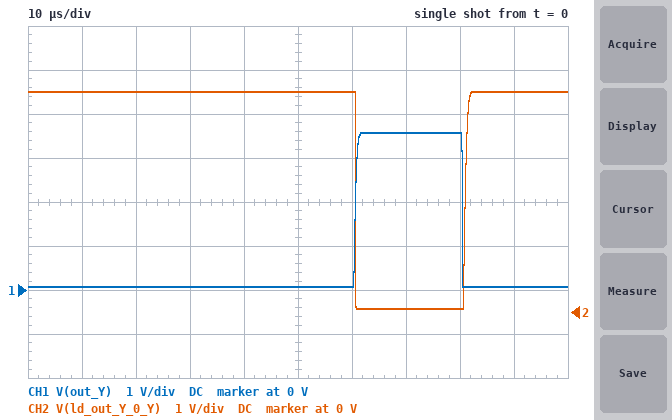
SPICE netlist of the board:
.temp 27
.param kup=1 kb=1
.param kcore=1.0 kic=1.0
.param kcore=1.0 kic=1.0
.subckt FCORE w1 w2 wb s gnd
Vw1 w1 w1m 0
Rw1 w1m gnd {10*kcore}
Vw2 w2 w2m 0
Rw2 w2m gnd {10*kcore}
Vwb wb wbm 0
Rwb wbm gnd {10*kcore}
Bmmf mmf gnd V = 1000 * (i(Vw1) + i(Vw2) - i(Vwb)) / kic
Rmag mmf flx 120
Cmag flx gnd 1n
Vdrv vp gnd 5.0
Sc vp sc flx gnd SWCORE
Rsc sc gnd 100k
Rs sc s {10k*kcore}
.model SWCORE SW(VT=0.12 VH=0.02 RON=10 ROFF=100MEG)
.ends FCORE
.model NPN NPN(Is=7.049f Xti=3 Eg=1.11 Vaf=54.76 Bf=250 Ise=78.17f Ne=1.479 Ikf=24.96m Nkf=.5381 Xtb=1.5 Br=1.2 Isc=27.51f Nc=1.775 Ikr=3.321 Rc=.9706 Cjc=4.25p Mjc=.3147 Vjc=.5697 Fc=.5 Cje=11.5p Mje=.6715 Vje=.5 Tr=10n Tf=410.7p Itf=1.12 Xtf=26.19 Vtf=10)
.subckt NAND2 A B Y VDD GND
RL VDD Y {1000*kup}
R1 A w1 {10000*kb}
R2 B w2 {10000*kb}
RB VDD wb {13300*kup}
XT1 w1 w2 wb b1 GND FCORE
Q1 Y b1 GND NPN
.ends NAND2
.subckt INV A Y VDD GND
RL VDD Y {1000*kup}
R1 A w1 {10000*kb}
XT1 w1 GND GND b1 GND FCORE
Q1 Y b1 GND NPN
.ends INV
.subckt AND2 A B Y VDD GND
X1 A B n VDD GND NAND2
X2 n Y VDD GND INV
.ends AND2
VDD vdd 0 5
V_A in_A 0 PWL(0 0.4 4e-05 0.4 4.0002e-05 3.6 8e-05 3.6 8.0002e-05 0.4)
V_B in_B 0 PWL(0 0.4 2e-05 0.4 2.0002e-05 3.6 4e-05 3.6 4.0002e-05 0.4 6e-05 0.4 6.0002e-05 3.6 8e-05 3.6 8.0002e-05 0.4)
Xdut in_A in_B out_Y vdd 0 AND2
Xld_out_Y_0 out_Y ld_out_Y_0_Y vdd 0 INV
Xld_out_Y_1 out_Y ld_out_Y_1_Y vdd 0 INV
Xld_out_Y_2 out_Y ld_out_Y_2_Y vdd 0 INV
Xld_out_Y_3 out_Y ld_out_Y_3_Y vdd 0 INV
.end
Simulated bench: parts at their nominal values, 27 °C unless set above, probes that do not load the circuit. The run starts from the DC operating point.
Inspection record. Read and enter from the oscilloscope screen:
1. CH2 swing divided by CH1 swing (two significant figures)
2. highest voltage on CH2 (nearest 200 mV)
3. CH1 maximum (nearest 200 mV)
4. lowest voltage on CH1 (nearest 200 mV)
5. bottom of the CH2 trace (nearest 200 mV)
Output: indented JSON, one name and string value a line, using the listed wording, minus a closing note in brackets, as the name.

{
  "CH2 swing divided by CH1 swing": "1.4",
  "highest voltage on CH2": "5.0 V",
  "CH1 maximum": "3.6 V",
  "lowest voltage on CH1": "0 V",
  "bottom of the CH2 trace": "0 V"
}
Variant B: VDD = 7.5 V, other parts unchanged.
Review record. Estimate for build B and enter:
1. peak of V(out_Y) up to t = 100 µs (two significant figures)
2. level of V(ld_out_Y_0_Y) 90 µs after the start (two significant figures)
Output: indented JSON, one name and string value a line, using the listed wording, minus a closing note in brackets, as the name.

{
  "peak of V(out_Y) up to t = 100 µs": "5.4 V",
  "level of V(ld_out_Y_0_Y) 90 µs after the start": "7.5 V"
}
